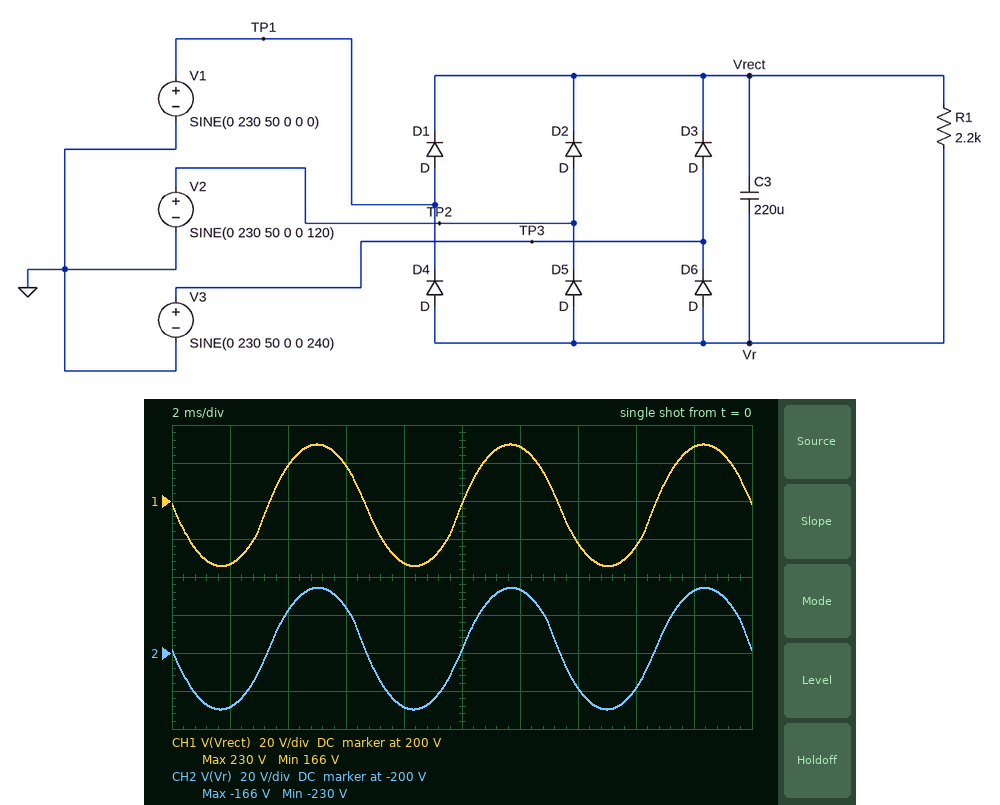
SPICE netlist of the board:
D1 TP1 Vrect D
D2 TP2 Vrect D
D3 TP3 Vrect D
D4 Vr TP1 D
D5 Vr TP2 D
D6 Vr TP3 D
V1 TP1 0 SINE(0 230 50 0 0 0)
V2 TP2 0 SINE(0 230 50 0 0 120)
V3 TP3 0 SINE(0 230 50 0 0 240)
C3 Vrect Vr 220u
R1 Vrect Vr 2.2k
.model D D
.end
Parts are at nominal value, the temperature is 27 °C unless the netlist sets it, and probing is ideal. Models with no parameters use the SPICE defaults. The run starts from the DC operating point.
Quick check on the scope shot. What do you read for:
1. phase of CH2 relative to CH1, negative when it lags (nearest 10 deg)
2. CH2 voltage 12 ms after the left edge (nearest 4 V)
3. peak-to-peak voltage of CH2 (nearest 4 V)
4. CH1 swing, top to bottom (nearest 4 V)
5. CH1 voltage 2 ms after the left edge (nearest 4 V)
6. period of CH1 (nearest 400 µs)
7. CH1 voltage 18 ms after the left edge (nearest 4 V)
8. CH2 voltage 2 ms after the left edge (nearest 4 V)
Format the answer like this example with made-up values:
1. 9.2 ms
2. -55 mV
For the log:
1. 0 deg
2. -168 V
3. 64 V
4. 64 V
5. 168 V
6. 6.8 ms
7. 228 V
8. -228 V
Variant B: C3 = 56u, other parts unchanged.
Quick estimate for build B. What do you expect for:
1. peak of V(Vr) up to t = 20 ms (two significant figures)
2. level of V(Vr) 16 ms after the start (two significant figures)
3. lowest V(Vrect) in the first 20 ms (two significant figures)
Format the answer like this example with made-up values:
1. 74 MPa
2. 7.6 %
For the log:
1. -160 V
2. -220 V
3. 160 V
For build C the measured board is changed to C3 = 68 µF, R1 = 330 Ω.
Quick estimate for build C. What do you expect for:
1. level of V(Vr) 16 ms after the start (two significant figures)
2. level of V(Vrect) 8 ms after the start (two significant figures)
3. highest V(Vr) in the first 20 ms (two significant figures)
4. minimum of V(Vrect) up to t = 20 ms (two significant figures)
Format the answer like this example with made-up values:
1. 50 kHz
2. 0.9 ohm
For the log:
1. -220 V
2. 150 V
3. -140 V
4. 140 V
